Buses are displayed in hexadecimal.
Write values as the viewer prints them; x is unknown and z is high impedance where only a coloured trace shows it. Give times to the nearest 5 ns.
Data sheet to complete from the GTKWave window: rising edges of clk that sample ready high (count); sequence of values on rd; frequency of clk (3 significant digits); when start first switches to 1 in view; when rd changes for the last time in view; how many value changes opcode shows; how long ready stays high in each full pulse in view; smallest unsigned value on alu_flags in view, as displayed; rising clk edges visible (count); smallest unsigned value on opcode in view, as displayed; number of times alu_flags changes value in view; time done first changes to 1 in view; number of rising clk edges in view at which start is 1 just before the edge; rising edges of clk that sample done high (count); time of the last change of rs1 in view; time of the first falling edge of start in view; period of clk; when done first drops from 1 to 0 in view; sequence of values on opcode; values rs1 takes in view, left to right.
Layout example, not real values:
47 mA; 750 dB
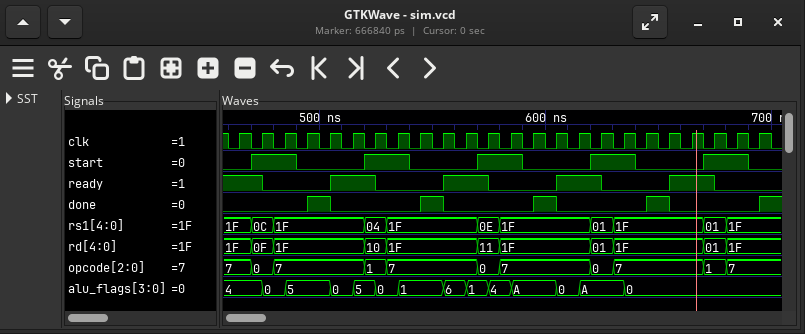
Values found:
10; 1F, 0F, 1F, 10, 1F, 11, 1F, 01, 1F, 01, 1F; 100 MHz; 470 ns; 680 ns; 10; 20 ns, 20 ns, 20 ns, 20 ns; 0; 24; 0; 13; 495 ns; 10; 4; 680 ns; 490 ns; 10 ns; 505 ns; 7, 0, 7, 1, 7, 0, 7, 0, 7, 1, 7; 1F, 0C, 1F, 04, 1F, 0E, 1F, 01, 1F, 01, 1F
